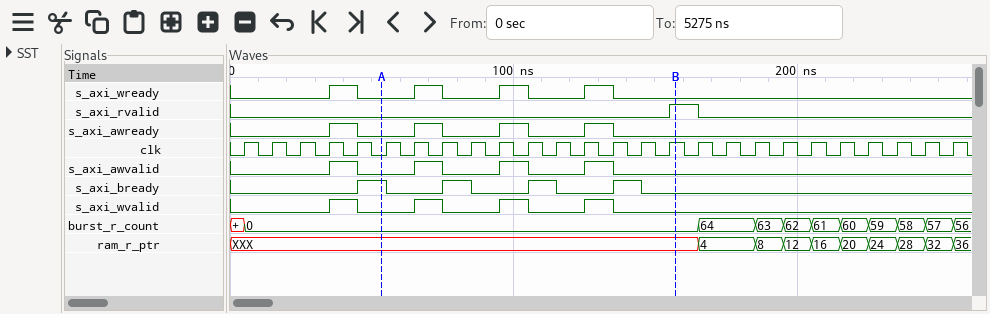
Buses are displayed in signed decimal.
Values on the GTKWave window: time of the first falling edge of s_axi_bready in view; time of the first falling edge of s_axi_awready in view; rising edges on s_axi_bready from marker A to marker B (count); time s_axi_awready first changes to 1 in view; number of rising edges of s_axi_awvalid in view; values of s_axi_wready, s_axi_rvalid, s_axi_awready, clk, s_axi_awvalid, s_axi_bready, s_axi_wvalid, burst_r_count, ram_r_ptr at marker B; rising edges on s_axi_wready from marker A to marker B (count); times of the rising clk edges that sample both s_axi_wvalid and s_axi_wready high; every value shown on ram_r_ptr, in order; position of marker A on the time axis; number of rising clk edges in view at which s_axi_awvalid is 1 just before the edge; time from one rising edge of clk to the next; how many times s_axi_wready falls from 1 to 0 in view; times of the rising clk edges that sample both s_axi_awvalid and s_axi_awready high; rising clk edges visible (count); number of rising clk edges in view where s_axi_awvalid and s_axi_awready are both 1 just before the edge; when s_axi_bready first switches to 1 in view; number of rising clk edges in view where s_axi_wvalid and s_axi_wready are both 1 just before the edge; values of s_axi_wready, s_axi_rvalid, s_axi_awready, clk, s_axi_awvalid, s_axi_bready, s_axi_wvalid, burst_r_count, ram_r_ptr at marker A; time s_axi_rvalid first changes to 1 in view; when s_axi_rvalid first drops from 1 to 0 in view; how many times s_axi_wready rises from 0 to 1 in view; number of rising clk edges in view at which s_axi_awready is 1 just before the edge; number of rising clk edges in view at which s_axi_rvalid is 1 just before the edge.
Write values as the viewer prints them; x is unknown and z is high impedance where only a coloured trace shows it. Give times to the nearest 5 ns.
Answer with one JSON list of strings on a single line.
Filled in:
["55 ns", "45 ns", "3", "35 ns", "4", "s_axi_wready=0, s_axi_rvalid=1, s_axi_awready=0, clk=1, s_axi_awvalid=0, s_axi_bready=0, s_axi_wvalid=0, burst_r_count=0, ram_r_ptr=XXX", "3", "45 ns, 75 ns, 105 ns, 135 ns", "XXX, 4, 8, 12, 16, 20, 24, 28, 32, 36", "55 ns", "4", "10 ns", "4", "45 ns, 75 ns, 105 ns, 135 ns", "26", "4", "45 ns", "4", "s_axi_wready=0, s_axi_rvalid=0, s_axi_awready=0, clk=0, s_axi_awvalid=0, s_axi_bready=1, s_axi_wvalid=0, burst_r_count=0, ram_r_ptr=XXX", "155 ns", "165 ns", "4", "4", "1"]
